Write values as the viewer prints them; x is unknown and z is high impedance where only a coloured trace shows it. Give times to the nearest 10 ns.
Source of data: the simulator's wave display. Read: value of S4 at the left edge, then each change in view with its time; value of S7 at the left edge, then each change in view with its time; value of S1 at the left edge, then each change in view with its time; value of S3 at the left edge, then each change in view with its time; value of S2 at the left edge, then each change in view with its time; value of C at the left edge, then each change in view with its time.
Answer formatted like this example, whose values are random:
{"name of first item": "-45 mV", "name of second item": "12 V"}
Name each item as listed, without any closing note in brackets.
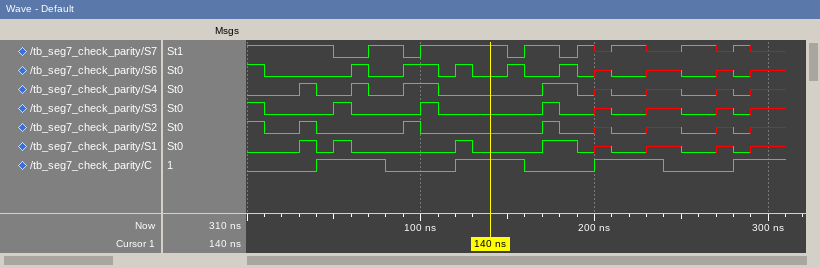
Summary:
{"value of S4 at the left edge, then each change in view with its time": "0, 1 at 30 ns, 0 at 40 ns, 1 at 60 ns, 0 at 70 ns, 1 at 90 ns, 0 at 110 ns, 1 at 170 ns, 0 at 190 ns, x at 200 ns, 0 at 210 ns, x at 230 ns, 0 at 250 ns, x at 270 ns, 0 at 280 ns, x at 290 ns", "value of S7 at the left edge, then each change in view with its time": "1, 0 at 50 ns, 1 at 70 ns, 0 at 90 ns, 1 at 100 ns, 0 at 150 ns, 1 at 160 ns, 0 at 180 ns, 1 at 190 ns, x at 200 ns, 1 at 210 ns, x at 230 ns, 1 at 250 ns, x at 270 ns, 1 at 280 ns, x at 290 ns", "value of S1 at the left edge, then each change in view with its time": "0, 1 at 30 ns, 0 at 40 ns, 1 at 50 ns, 0 at 60 ns, 1 at 120 ns, 0 at 130 ns, 1 at 170 ns, 0 at 190 ns, x at 200 ns, 0 at 210 ns, x at 230 ns, 0 at 250 ns, x at 270 ns, 0 at 280 ns, x at 290 ns", "value of S3 at the left edge, then each change in view with its time": "1, 0 at 10 ns, 1 at 50 ns, 0 at 60 ns, 1 at 100 ns, 0 at 110 ns, 1 at 170 ns, 0 at 180 ns, x at 200 ns, 0 at 210 ns, x at 230 ns, 0 at 250 ns, x at 270 ns, 0 at 280 ns, x at 290 ns", "value of S2 at the left edge, then each change in view with its time": "1, 0 at 10 ns, 1 at 30 ns, 0 at 40 ns, 1 at 90 ns, 0 at 100 ns, 1 at 170 ns, 0 at 180 ns, x at 200 ns, 0 at 210 ns, x at 230 ns, 0 at 250 ns, x at 270 ns, 0 at 280 ns, x at 290 ns", "value of C at the left edge, then each change in view with its time": "0, 1 at 40 ns, 0 at 80 ns, 1 at 120 ns, 0 at 160 ns, 1 at 200 ns, 0 at 240 ns, 1 at 280 ns"}
